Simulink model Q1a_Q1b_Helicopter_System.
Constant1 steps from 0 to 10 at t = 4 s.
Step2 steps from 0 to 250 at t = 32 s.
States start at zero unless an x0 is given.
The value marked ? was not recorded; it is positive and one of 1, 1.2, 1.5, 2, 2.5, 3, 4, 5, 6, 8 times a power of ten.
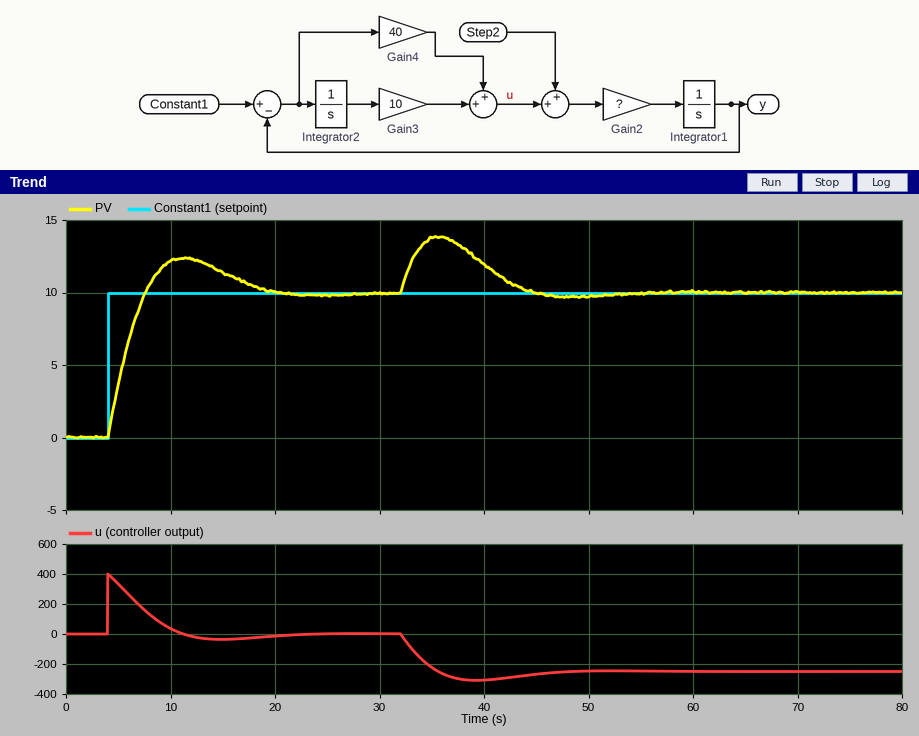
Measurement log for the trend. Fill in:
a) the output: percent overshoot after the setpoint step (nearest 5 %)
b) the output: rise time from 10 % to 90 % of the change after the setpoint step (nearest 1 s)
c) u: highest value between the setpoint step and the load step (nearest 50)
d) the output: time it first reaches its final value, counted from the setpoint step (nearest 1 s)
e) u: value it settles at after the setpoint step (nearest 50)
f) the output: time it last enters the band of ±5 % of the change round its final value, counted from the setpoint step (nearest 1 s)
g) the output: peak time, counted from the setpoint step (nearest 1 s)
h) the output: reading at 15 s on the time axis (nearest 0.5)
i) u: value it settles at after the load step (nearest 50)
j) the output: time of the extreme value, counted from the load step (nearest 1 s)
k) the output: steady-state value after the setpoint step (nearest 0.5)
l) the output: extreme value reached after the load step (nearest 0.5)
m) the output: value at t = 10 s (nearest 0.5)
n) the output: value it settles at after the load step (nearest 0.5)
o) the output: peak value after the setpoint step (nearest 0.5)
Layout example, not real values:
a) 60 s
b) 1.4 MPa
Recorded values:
a) 25 %
b) 3 s
c) 400
d) 4 s
e) 0
f) 14 s
g) 7 s
h) 11.5
i) -250
j) 4 s
k) 10.0
l) 14.0
m) 12.0
n) 10.0
o) 12.5
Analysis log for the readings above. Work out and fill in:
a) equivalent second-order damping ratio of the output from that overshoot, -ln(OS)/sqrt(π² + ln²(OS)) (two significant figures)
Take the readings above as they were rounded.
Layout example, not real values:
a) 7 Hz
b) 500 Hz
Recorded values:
a) 0.40
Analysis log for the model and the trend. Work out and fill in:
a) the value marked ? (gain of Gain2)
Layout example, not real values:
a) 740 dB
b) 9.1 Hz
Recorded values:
a) 0.01
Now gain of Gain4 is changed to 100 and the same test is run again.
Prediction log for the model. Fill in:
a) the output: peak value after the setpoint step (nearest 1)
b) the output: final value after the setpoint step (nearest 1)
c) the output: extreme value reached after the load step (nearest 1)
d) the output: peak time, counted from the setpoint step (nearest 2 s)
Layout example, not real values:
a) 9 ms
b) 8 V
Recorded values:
a) 11
b) 10
c) 12
d) 6 s
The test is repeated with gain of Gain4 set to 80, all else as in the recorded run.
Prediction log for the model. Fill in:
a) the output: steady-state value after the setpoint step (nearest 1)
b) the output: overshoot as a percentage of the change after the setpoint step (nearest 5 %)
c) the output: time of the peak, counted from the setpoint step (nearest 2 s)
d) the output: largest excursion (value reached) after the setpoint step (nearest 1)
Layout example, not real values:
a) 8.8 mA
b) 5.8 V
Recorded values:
a) 10
b) 10 %
c) 6 s
d) 11
